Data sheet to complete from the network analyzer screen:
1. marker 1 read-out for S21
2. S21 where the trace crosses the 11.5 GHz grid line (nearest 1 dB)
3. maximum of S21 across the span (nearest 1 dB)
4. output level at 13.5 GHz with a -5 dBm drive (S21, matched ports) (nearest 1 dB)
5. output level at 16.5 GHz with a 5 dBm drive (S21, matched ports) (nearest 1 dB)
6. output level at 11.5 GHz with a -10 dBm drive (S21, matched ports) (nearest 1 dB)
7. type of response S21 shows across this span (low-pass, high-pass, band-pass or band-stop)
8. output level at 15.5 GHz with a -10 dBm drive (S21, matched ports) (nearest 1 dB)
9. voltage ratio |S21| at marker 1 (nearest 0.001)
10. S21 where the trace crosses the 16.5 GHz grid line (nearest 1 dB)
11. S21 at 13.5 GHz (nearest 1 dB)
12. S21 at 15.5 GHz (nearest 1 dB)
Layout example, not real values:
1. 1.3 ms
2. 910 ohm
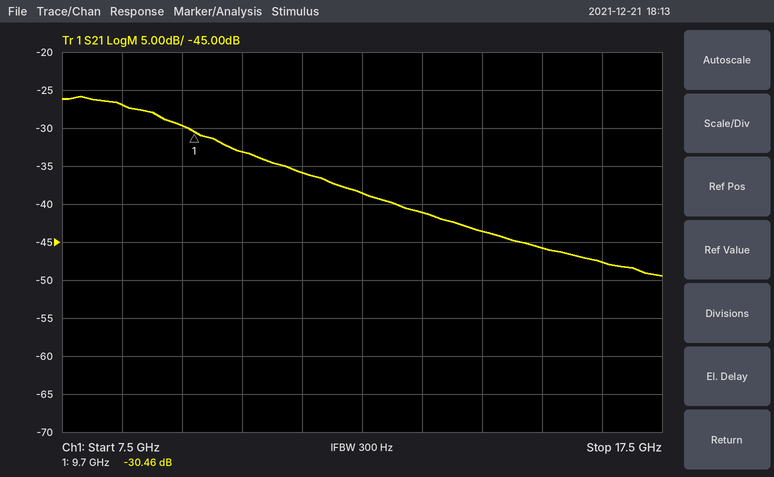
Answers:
1. -30.46 dB
2. -36 dB
3. -26 dB
4. -46 dBm
5. -43 dBm
6. -46 dBm
7. low-pass
8. -56 dBm
9. 0.030
10. -48 dB
11. -41 dB
12. -46 dB
